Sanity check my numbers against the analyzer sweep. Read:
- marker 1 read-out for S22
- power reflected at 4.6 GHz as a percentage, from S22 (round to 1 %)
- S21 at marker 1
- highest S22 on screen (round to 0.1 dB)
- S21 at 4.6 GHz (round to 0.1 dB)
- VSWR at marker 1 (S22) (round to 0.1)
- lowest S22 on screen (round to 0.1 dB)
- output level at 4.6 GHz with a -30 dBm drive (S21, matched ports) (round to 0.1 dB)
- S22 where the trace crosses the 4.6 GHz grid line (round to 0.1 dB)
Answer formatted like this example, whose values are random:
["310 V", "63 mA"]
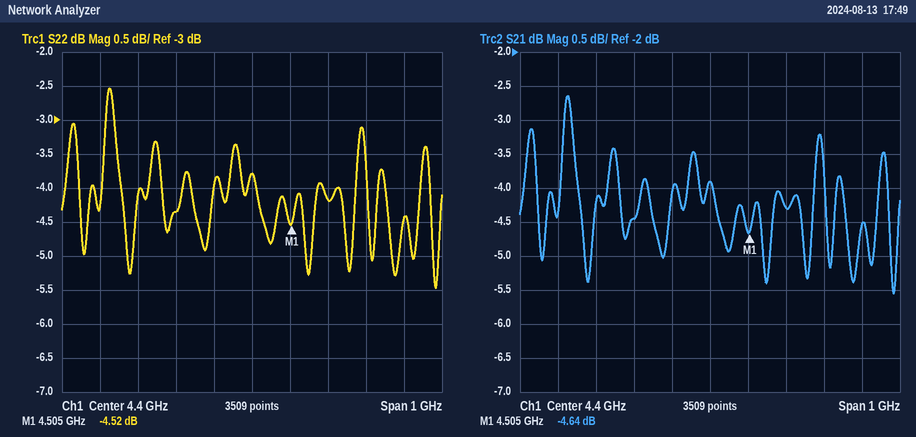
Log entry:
["-4.52 dB", "38 %", "-4.64 dB", "-2.5 dB", "-4.3 dB", "3.9", "-5.5 dB", "-34.3 dBm", "-4.2 dB"]
